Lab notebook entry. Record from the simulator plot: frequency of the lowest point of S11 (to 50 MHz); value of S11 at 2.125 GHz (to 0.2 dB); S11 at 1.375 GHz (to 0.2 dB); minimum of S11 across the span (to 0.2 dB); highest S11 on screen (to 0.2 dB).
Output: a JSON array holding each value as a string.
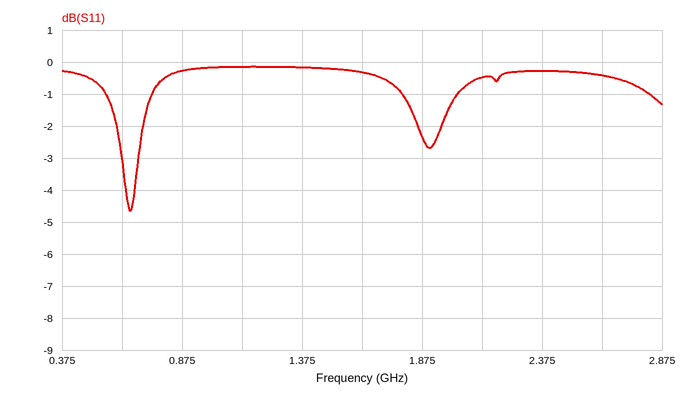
["650 MHz", "-0.4 dB", "-0.2 dB", "-4.6 dB", "-0.2 dB"]
